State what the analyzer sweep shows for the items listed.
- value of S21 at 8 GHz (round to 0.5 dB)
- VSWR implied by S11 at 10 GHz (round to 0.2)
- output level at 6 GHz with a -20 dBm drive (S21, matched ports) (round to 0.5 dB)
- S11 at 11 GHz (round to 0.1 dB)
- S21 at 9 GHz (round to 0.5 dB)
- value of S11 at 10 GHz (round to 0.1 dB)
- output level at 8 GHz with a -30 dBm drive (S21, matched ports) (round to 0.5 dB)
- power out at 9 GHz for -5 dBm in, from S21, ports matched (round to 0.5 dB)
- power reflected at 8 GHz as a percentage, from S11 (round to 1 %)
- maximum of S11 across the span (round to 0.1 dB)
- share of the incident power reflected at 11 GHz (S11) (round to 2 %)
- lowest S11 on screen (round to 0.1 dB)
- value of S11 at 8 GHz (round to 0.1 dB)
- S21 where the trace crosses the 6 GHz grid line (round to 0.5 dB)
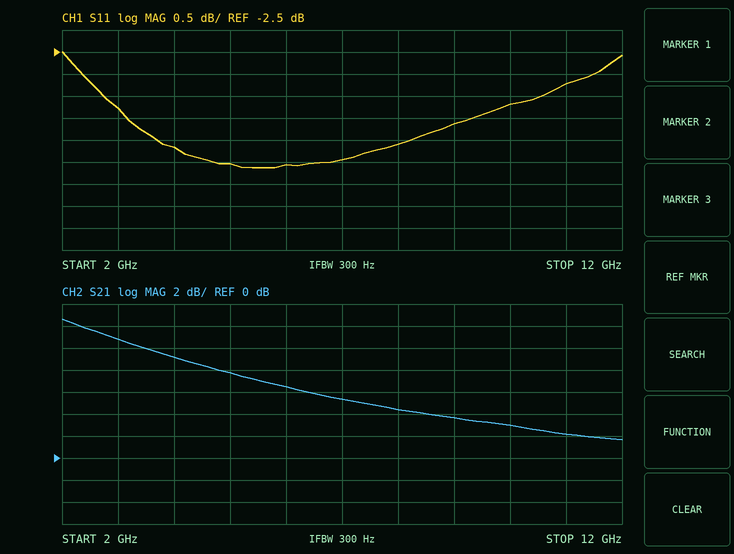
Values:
4.5 dB
4.8
-13.5 dBm
-3.2 dB
3.5 dB
-3.7 dB
-25.5 dBm
-1.5 dBm
35 %
-2.5 dB
48 %
-5.1 dB
-4.6 dB
6.5 dB
